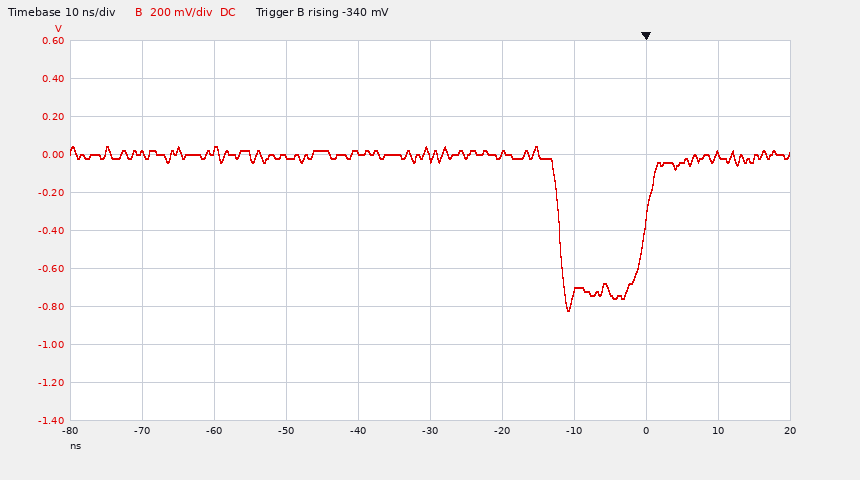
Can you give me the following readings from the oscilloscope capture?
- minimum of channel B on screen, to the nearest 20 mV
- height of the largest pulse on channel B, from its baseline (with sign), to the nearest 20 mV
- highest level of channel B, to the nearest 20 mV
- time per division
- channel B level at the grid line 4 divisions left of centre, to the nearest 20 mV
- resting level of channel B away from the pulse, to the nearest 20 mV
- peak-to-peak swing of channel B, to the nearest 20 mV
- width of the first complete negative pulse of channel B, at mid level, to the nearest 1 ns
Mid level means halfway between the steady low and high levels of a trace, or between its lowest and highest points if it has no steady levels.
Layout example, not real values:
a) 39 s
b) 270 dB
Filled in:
a) -820 mV
b) -820 mV
c) 40 mV
d) 10 ns
e) 0 mV
f) 0 mV
g) 860 mV
h) 12 ns
